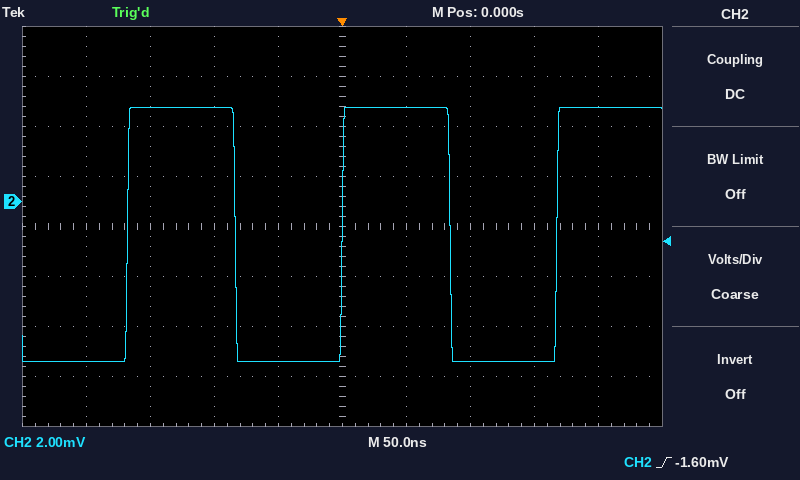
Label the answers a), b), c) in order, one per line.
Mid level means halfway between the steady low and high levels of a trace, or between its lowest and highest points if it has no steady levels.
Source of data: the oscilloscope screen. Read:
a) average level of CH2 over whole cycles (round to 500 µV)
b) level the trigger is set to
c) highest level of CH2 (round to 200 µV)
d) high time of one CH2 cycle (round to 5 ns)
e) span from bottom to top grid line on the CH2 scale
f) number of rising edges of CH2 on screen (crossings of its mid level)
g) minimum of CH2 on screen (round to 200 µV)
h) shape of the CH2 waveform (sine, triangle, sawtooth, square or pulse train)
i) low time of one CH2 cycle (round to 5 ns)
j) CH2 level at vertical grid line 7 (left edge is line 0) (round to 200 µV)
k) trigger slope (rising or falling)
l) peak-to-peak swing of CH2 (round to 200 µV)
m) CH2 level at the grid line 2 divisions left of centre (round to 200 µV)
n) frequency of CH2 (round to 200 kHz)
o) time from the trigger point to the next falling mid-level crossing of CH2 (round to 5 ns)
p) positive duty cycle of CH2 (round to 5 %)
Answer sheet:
a) -1.5 mV
b) -1.60 mV
c) 3.8 mV
d) 85 ns
e) 16 mV
f) 3
g) -6.4 mV
h) square
i) 85 ns
j) -6.4 mV
k) rising
l) 10.2 mV
m) 3.8 mV
n) 6.0 MHz
o) 85 ns
p) 50 %
